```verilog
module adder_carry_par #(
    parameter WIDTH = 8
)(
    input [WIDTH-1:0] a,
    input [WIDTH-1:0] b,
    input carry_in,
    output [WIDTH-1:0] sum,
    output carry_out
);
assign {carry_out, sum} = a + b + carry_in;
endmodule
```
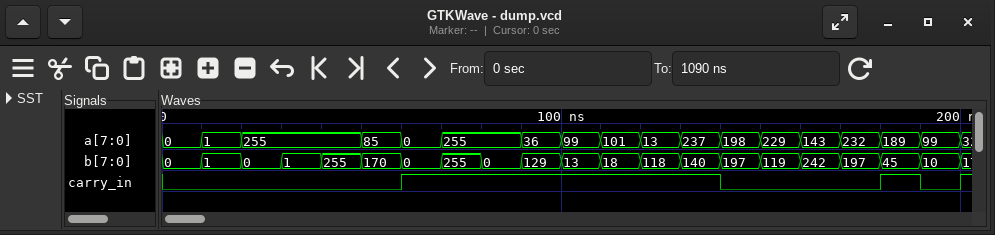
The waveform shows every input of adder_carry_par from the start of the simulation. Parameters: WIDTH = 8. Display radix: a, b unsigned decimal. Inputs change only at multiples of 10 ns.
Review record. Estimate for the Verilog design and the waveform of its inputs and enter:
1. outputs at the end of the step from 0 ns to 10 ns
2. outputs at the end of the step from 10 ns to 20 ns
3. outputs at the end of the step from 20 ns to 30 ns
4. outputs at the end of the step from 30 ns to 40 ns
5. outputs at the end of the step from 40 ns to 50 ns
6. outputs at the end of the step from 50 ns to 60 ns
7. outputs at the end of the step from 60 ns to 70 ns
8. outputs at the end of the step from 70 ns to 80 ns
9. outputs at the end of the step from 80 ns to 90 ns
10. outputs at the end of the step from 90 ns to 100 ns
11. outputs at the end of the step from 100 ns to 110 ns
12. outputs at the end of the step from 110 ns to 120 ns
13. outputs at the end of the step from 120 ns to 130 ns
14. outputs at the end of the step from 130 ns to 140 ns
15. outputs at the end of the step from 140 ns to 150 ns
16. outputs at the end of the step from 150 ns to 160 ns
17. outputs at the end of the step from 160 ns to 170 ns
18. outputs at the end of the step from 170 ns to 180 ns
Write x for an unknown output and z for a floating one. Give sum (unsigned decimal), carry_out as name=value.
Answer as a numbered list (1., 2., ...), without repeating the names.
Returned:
1. sum=0, carry_out=0
2. sum=2, carry_out=0
3. sum=255, carry_out=0
4. sum=0, carry_out=1
5. sum=254, carry_out=1
6. sum=255, carry_out=0
7. sum=1, carry_out=0
8. sum=255, carry_out=1
9. sum=0, carry_out=1
10. sum=166, carry_out=0
11. sum=113, carry_out=0
12. sum=120, carry_out=0
13. sum=132, carry_out=0
14. sum=122, carry_out=1
15. sum=139, carry_out=1
16. sum=92, carry_out=1
17. sum=129, carry_out=1
18. sum=173, carry_out=1
